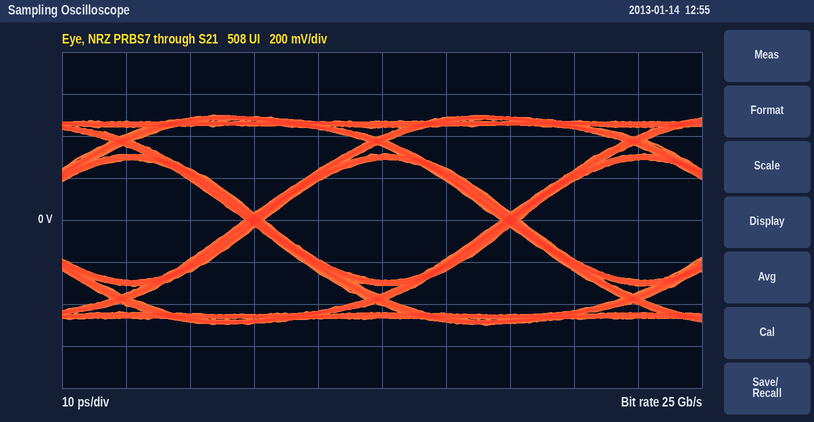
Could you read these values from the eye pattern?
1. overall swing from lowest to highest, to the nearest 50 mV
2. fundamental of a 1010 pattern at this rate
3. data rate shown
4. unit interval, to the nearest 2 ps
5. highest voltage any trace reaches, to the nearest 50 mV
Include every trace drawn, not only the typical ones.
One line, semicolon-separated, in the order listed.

1.00 V; 12.5 GHz; 25 Gb/s; 40 ps; 500 mV
